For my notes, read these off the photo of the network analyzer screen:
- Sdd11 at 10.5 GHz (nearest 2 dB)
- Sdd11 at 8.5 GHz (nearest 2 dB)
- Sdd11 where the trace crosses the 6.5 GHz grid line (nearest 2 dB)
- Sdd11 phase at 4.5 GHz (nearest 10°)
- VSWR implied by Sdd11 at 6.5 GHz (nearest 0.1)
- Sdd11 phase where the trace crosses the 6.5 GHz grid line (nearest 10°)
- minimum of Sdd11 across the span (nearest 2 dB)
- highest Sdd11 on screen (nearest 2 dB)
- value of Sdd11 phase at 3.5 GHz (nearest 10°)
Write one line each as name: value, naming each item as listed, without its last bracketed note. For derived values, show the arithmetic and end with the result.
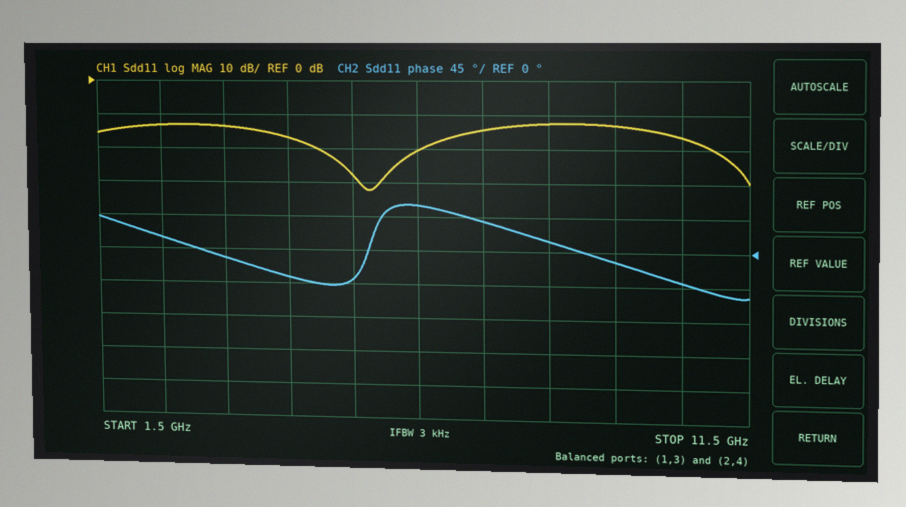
Sdd11 at 10.5 GHz: -16 dB
Sdd11 at 8.5 GHz: -12 dB
Sdd11 where the trace crosses the 6.5 GHz grid line: -20 dB
Sdd11 phase at 4.5 GHz: -40°
VSWR implied by Sdd11 at 6.5 GHz: |Γ| = 10^(-20/20) = 0.1000; VSWR = (1 + 0.1000)/(1 − 0.1000) ≈ 1.2
Sdd11 phase where the trace crosses the 6.5 GHz grid line: 60°
minimum of Sdd11 across the span: -32 dB
highest Sdd11 on screen: -12 dB
value of Sdd11 phase at 3.5 GHz: -10°
